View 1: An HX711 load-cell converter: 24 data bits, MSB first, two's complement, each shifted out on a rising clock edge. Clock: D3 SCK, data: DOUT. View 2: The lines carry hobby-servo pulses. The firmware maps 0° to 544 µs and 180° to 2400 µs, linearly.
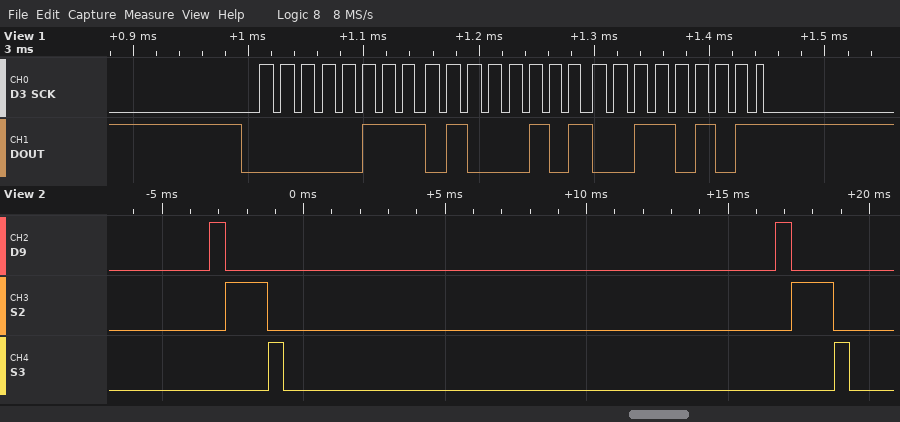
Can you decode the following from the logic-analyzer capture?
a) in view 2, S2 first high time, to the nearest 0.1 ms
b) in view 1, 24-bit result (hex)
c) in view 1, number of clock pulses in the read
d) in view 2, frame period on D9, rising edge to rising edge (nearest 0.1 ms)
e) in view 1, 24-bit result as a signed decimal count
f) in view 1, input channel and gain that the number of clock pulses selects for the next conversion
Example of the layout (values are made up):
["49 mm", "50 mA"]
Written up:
["1.5 ms", "0x074535", "25", "20.0 ms", "476469", "channel A, gain 128"]
